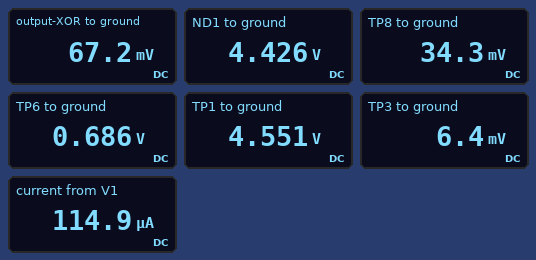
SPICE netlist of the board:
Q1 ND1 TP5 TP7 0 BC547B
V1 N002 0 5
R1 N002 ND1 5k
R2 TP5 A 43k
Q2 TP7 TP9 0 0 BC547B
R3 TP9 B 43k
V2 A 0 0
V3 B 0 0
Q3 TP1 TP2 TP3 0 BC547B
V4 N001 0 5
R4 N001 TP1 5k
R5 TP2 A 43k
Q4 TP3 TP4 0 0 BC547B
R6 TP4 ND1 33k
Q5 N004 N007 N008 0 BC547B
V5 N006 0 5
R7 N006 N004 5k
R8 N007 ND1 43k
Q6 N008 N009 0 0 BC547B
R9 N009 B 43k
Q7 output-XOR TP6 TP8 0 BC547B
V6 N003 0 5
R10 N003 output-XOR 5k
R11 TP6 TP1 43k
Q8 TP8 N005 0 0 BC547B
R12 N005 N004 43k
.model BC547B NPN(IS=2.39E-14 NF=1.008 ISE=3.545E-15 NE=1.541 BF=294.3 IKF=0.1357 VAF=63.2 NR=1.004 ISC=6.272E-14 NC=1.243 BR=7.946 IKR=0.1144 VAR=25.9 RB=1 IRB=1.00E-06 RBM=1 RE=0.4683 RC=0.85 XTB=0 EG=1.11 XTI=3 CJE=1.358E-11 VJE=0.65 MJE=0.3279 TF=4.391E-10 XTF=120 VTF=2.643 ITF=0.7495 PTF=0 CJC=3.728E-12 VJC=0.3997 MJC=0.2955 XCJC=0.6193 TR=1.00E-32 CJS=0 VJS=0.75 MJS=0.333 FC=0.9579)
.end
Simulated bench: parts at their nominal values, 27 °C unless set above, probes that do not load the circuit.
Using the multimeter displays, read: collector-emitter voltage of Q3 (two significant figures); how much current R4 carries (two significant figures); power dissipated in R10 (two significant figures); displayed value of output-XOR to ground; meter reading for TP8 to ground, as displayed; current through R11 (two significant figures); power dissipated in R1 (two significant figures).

4.5 V
90 µA
4.9 mW
67.2 mV
34.3 mV
90 µA
66 µW
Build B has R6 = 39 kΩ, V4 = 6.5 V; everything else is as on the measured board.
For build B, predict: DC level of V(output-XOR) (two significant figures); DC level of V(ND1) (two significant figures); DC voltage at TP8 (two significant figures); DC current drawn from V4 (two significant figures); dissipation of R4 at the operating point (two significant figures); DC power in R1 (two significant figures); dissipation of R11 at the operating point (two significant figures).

63 mV
4.5 V
35 mV
120 µA
73 µW
49 µW
630 µW
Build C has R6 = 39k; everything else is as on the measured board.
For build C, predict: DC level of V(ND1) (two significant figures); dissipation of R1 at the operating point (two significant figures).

4.5 V
49 µW
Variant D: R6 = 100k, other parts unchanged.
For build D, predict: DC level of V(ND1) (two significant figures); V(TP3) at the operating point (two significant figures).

4.8 V
6.3 mV
